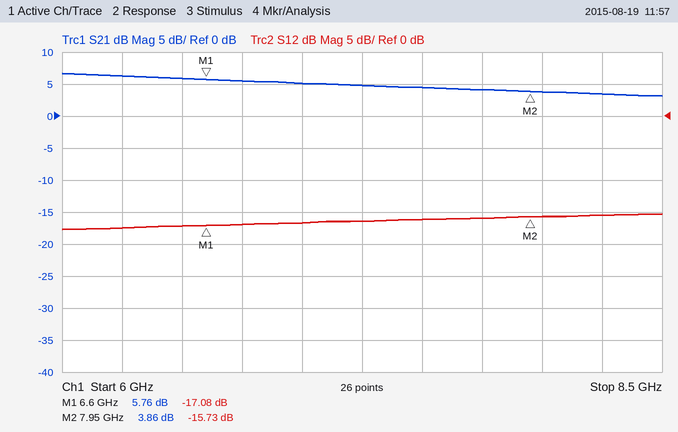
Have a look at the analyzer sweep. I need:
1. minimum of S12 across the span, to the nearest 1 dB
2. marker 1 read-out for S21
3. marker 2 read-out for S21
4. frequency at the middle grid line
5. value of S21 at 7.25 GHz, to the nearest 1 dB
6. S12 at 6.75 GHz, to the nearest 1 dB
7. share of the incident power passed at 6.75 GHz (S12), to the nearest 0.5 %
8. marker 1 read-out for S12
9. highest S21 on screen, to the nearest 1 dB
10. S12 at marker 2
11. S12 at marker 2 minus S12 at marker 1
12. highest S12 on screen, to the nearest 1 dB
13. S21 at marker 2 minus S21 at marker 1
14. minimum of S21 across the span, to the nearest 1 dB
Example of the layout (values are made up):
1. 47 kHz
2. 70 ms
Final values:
1. -18 dB
2. 5.76 dB
3. 3.86 dB
4. 7.25 GHz
5. 5 dB
6. -17 dB
7. 2.0 %
8. -17.08 dB
9. 7 dB
10. -15.73 dB
11. 1.35 dB
12. -15 dB
13. -1.90 dB
14. 3 dB
